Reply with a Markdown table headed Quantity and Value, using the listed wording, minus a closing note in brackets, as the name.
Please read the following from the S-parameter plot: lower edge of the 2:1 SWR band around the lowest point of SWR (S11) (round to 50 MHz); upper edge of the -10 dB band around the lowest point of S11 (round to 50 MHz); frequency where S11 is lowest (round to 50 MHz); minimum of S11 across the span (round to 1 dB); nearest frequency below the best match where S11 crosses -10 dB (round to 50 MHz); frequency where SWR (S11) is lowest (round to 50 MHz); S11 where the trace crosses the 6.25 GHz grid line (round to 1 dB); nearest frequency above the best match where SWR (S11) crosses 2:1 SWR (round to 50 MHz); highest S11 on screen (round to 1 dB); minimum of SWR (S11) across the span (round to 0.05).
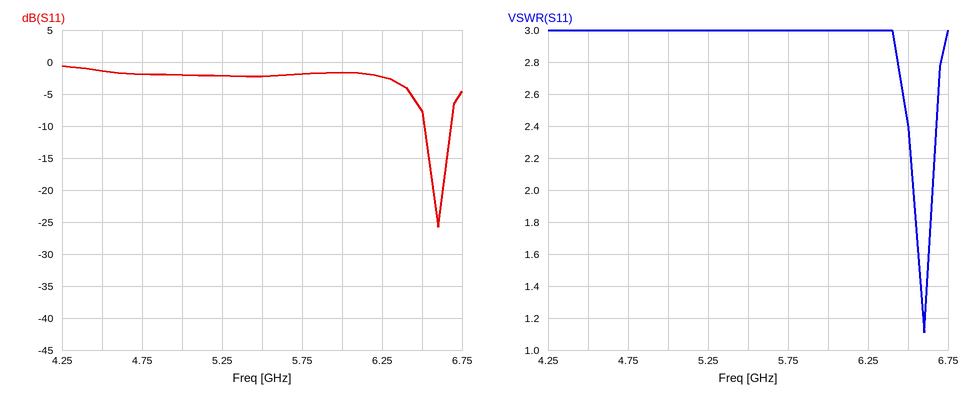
| Quantity | Value |
|---|---|
| lower edge of the 2:1 SWR band around the lowest point of SWR (S11) | 6.55 GHz |
| upper edge of the -10 dB band around the lowest point of S11 | 6.70 GHz |
| frequency where S11 is lowest | 6.60 GHz |
| minimum of S11 across the span | -26 dB |
| nearest frequency below the best match where S11 crosses -10 dB | 6.50 GHz |
| frequency where SWR (S11) is lowest | 6.60 GHz |
| S11 where the trace crosses the 6.25 GHz grid line | -2 dB |
| nearest frequency above the best match where SWR (S11) crosses 2:1 SWR | 6.65 GHz |
| highest S11 on screen | -1 dB |
| minimum of SWR (S11) across the span | 1.10 |
